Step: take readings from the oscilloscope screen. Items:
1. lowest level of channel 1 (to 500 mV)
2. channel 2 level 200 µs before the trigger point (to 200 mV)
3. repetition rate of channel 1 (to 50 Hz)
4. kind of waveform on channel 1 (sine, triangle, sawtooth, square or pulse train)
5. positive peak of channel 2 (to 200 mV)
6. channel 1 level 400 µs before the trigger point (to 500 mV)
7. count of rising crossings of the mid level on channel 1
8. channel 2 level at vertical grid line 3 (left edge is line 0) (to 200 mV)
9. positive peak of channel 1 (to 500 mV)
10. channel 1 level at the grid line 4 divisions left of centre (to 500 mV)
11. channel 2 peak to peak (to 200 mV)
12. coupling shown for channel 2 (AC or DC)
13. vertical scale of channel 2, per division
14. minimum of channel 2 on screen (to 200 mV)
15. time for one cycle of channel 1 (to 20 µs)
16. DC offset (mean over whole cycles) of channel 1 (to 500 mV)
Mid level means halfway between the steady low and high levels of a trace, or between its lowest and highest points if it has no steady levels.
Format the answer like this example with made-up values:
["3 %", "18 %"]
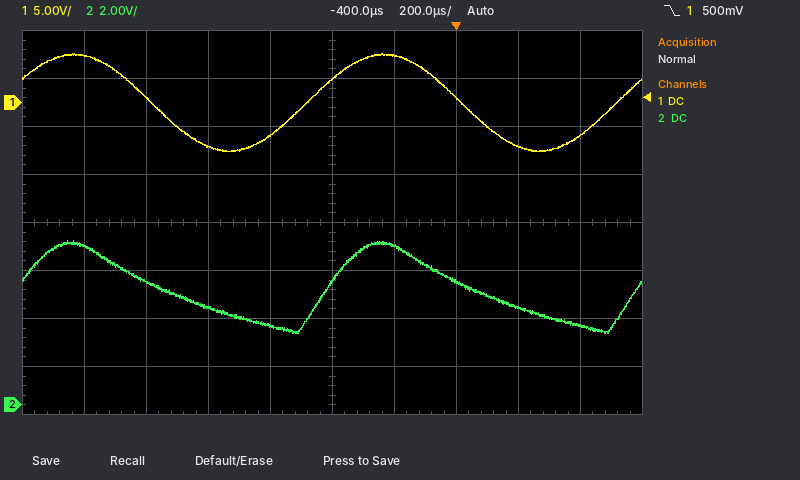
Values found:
["-5.0 V", "6.6 V", "1.00 kHz", "sine", "6.8 V", "2.5 V", "2", "4.0 V", "5.0 V", "5.0 V", "3.8 V", "DC", "2 V", "3.0 V", "1.00 ms", "0.0 V"]
